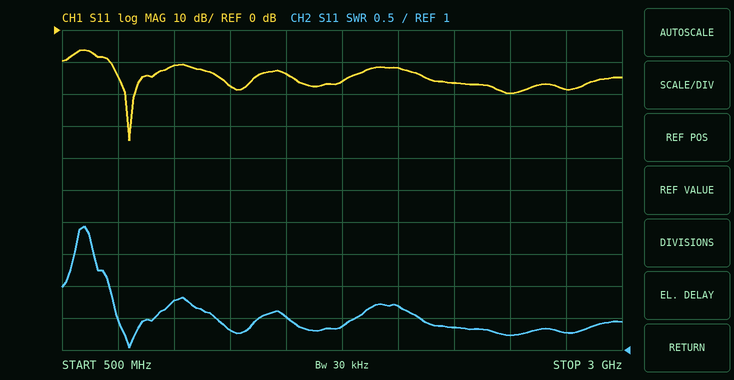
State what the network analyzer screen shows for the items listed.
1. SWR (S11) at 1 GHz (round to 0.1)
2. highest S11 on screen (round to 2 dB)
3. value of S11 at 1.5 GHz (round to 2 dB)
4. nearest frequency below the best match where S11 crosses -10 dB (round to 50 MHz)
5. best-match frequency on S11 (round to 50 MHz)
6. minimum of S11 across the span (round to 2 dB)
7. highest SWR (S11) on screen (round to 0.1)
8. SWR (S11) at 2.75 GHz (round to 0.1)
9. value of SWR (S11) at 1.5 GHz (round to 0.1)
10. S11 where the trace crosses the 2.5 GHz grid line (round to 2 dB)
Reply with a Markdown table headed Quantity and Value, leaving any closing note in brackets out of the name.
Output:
| Quantity | Value |
|---|---|
| SWR (S11) at 1 GHz | 1.8 |
| highest S11 on screen | -6 dB |
| value of S11 at 1.5 GHz | -14 dB |
| nearest frequency below the best match where S11 crosses -10 dB | 700 MHz |
| best-match frequency on S11 | 800 MHz |
| minimum of S11 across the span | -34 dB |
| highest SWR (S11) on screen | 2.9 |
| SWR (S11) at 2.75 GHz | 1.3 |
| value of SWR (S11) at 1.5 GHz | 1.5 |
| S11 where the trace crosses the 2.5 GHz grid line | -20 dB |
